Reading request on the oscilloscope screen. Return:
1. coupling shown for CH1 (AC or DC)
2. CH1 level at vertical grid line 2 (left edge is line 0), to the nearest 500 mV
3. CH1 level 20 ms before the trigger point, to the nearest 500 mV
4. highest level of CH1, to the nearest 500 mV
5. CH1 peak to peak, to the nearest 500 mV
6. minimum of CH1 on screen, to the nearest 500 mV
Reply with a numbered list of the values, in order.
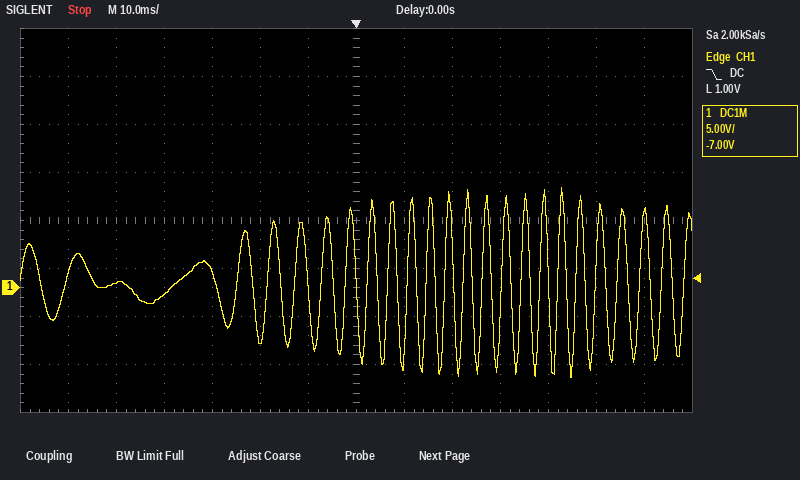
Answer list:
1. DC
2. 500 mV
3. -5.5 V
4. 10.5 V
5. 20.0 V
6. -9.5 V
